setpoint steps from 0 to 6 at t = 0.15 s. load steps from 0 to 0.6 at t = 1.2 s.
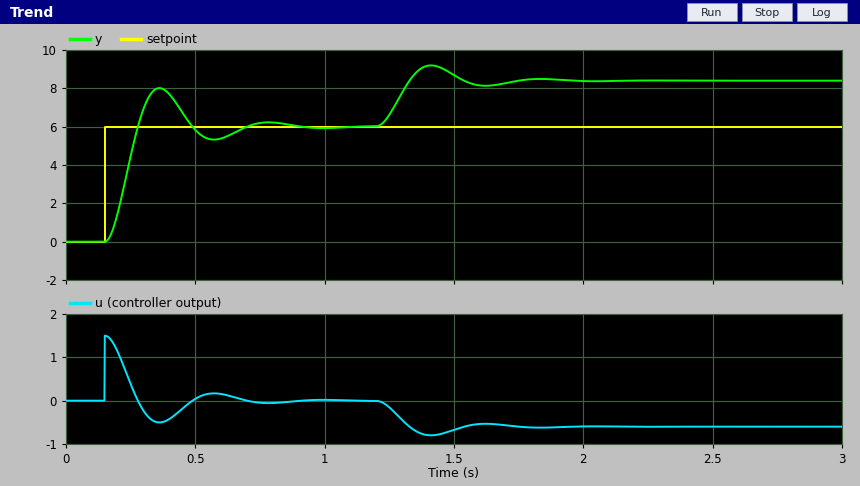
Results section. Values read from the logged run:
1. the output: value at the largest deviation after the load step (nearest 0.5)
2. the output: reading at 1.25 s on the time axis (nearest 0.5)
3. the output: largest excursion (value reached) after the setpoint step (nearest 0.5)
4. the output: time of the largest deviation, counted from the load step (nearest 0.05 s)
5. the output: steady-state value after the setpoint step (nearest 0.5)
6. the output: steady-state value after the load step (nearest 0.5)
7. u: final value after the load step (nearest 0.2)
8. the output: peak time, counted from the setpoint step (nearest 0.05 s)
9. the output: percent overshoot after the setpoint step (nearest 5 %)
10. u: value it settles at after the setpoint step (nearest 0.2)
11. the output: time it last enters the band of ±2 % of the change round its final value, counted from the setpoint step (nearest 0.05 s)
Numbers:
9.0
6.5
8.0
0.20 s
6.0
8.5
-0.6
0.20 s
35 %
0.0
0.70 s
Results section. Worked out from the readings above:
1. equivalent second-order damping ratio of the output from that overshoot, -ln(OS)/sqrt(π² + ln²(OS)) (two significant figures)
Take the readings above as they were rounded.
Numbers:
0.32
